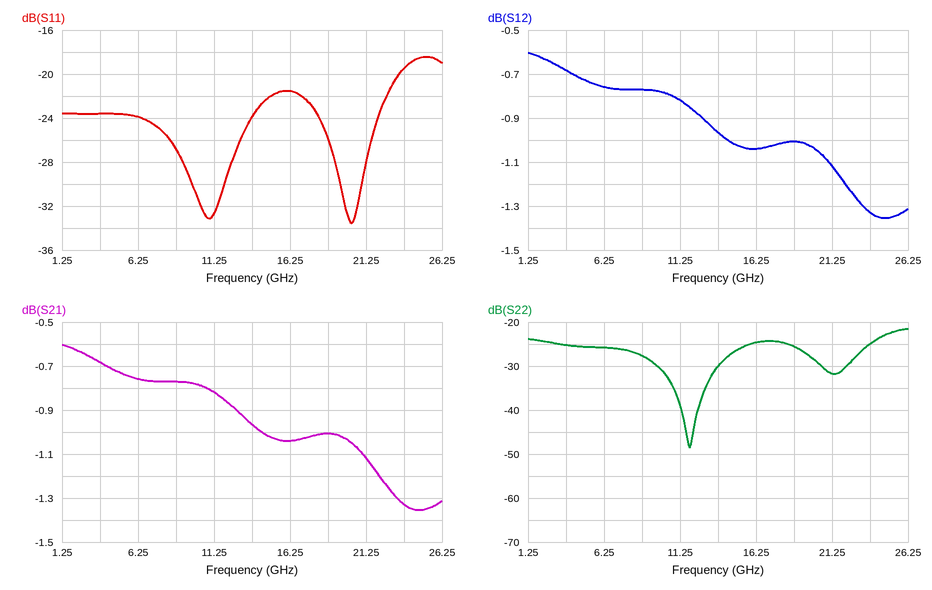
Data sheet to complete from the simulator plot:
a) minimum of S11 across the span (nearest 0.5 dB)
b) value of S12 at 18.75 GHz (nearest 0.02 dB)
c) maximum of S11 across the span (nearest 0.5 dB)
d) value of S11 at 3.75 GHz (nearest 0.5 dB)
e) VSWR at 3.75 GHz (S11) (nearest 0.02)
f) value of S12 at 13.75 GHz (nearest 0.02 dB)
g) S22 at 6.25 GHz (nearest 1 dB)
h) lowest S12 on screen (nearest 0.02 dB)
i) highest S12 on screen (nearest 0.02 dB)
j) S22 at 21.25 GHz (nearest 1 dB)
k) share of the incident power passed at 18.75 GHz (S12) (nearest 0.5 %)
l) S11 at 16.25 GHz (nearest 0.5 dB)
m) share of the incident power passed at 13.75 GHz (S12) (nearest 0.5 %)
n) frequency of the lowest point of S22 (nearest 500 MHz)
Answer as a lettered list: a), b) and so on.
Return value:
a) -33.5 dB
b) -1.00 dB
c) -18.5 dB
d) -23.5 dB
e) 1.14
f) -0.96 dB
g) -26 dB
h) -1.36 dB
i) -0.60 dB
j) -32 dB
k) 79.5 %
l) -21.5 dB
m) 80.0 %
n) 12.0 GHz
